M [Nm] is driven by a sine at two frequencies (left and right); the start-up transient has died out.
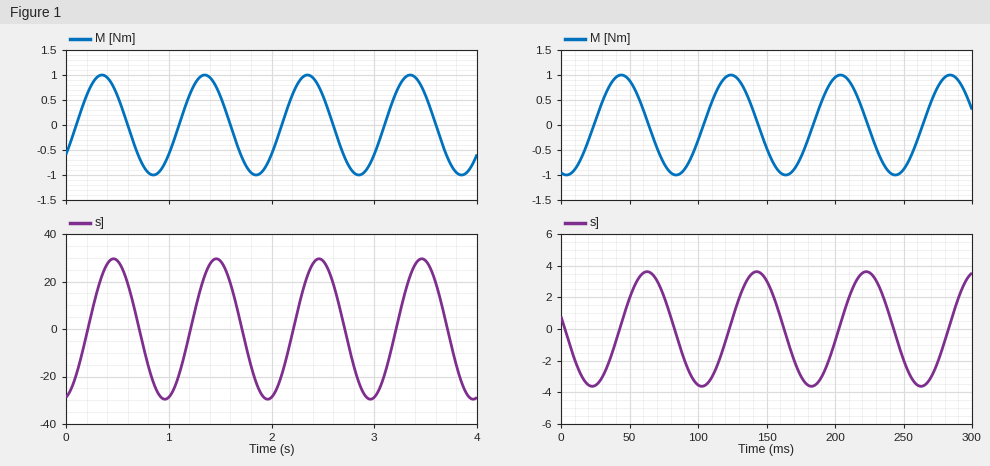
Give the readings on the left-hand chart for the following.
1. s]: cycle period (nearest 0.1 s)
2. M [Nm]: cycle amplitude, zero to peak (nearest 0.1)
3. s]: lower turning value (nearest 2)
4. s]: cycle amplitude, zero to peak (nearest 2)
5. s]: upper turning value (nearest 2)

1.0 s
1.0
-30
30
30
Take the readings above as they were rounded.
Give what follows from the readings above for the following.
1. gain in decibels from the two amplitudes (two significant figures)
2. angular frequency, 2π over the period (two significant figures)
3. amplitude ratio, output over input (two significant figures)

30 dB
6.3 rad/s
30
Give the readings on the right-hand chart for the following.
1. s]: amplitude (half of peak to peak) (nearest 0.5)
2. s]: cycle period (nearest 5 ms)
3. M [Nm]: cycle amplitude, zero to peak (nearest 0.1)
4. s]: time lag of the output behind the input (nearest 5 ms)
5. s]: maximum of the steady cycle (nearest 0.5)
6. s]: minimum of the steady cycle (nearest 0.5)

3.5
80 ms
1.0
20 ms
3.5
-3.5
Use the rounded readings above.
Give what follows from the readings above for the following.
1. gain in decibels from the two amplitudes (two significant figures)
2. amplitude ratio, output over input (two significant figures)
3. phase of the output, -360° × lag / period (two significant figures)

11 dB
3.5
-90°
